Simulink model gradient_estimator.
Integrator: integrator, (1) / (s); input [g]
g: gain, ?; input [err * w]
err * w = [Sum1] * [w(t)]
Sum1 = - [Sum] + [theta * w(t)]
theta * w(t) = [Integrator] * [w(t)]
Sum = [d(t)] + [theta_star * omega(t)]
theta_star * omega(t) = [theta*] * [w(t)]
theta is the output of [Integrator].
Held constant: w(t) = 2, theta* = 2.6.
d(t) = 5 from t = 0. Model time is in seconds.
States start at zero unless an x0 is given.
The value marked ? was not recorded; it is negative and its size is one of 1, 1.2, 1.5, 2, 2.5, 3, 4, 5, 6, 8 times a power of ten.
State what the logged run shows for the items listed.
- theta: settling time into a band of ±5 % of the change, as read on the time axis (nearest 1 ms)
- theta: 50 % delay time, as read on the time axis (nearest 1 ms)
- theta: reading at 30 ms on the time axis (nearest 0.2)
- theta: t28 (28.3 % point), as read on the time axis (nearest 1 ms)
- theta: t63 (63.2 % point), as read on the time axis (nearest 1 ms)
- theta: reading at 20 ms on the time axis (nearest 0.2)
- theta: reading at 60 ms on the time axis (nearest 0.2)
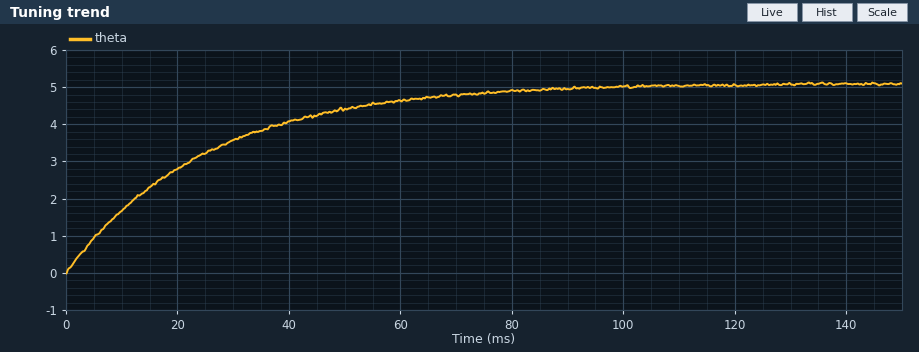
75 ms
17 ms
3.6
8 ms
25 ms
2.8
4.6
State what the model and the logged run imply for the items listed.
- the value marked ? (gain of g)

-10
